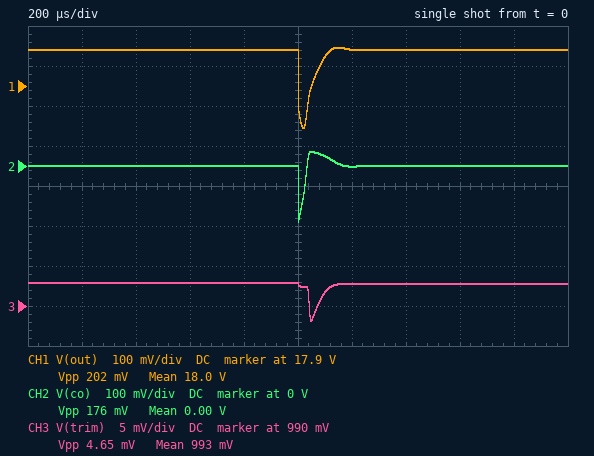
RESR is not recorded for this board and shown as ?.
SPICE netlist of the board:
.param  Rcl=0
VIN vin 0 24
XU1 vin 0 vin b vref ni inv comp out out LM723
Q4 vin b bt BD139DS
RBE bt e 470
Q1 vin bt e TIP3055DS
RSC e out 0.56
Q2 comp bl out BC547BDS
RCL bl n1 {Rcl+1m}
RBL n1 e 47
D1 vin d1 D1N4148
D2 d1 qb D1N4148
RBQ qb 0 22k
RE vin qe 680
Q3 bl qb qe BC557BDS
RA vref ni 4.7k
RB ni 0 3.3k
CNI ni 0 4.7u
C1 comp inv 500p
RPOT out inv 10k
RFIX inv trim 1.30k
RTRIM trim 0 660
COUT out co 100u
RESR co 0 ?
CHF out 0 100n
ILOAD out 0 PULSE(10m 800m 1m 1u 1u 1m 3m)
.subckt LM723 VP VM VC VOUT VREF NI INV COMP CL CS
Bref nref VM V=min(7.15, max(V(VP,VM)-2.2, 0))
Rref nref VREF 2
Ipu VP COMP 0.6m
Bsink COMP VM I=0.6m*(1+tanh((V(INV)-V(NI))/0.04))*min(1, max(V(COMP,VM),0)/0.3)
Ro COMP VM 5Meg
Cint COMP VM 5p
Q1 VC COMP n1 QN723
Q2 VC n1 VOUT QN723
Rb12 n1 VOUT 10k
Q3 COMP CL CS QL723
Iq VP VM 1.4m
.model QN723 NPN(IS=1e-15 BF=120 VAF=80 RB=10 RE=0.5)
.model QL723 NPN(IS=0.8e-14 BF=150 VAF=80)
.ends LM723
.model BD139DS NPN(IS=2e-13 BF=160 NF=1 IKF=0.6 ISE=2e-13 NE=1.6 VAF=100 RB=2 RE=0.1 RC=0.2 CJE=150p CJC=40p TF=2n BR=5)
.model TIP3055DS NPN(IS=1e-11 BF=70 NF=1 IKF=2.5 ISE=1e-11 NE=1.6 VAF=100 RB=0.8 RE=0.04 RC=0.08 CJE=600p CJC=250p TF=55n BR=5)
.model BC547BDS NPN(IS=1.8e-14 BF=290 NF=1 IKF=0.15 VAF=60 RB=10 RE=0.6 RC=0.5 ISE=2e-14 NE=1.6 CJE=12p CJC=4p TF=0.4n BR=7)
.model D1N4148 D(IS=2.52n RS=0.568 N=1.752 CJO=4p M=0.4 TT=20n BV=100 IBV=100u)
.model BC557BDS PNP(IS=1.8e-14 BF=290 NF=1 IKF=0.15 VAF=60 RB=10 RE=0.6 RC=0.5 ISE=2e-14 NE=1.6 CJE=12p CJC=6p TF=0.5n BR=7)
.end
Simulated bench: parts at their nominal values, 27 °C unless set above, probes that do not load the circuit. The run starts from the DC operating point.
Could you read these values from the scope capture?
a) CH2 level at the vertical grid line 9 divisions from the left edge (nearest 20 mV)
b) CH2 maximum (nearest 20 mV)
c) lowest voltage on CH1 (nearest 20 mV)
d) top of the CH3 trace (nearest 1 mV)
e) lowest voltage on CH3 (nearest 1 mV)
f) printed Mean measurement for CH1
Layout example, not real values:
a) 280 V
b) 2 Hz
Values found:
a) 0 V
b) 40 mV
c) 17.80 V
d) 993 mV
e) 988 mV
f) 18.0 V
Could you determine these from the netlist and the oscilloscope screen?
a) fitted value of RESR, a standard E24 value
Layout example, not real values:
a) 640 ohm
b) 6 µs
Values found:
a) 0.18 Ω
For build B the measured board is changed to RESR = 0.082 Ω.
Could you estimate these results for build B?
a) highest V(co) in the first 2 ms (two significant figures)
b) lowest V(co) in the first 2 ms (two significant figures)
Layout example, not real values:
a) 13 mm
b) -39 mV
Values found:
a) 18 mV
b) -64 mV
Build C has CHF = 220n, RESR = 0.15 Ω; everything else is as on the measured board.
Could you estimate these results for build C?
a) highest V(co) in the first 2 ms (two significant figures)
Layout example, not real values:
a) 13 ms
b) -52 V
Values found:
a) 31 mV
